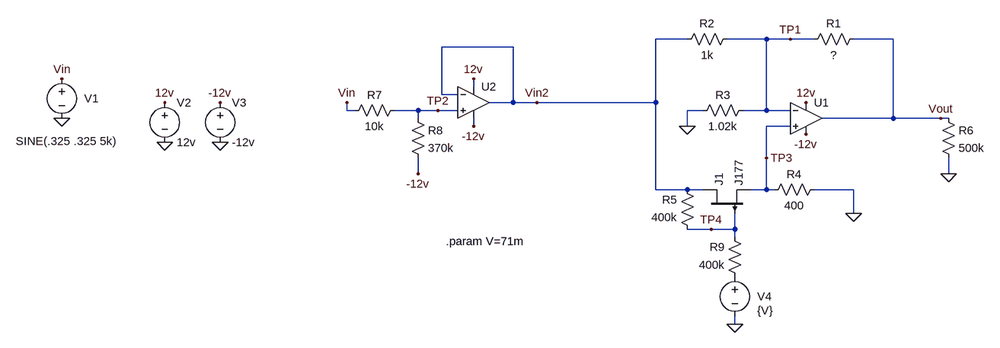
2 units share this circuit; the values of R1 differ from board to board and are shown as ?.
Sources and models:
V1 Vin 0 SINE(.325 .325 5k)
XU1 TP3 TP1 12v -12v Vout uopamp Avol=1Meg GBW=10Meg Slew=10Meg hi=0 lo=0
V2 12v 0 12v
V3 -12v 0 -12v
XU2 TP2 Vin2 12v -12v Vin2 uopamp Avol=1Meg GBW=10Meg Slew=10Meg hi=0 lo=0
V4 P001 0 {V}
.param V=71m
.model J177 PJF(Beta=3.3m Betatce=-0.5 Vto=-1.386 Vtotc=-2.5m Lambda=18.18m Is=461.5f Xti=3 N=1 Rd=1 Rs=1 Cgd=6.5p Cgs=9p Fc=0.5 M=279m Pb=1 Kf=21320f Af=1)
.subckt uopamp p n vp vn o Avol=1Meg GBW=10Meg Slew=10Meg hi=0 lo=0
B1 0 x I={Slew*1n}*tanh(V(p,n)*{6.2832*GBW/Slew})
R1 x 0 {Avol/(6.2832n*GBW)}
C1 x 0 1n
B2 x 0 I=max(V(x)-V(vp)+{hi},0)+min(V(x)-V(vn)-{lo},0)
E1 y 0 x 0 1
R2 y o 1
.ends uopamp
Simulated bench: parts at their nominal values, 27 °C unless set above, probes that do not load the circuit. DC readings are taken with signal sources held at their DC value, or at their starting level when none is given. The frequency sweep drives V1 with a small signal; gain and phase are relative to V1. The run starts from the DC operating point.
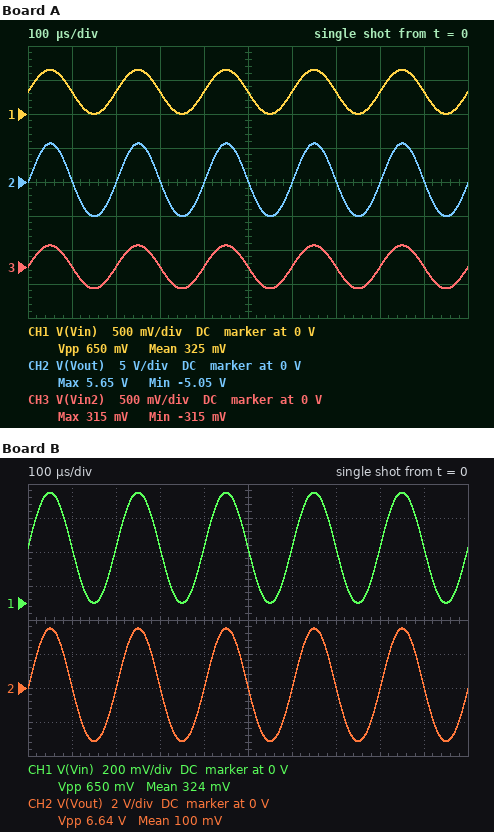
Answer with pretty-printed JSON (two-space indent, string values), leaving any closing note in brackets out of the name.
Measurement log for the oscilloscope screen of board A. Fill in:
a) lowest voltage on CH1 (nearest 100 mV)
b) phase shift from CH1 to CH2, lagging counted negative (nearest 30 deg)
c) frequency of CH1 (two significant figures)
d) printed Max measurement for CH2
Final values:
{
  "lowest voltage on CH1": "0 V",
  "phase shift from CH1 to CH2, lagging counted negative": "0 deg",
  "frequency of CH1": "5.0 kHz",
  "printed Max measurement for CH2": "5.65 V"
}
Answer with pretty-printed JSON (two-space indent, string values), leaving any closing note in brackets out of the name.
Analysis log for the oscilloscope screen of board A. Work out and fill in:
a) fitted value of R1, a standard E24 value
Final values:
{
  "fitted value of R1, a standard E24 value": "30 kΩ"
}
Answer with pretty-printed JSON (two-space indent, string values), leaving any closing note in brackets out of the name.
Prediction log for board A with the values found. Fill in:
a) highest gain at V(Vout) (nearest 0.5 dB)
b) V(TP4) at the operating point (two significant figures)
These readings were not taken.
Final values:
{
  "highest gain at V(Vout)": "24.5 dB",
  "V(TP4) at the operating point": "36 mV"
}
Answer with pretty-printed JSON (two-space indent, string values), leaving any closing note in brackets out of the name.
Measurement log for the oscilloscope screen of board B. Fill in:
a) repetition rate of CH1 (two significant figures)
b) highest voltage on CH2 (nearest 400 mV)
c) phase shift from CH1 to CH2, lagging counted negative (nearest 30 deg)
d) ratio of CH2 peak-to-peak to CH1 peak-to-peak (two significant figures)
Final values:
{
  "repetition rate of CH1": "5.0 kHz",
  "highest voltage on CH2": "3.6 V",
  "phase shift from CH1 to CH2, lagging counted negative": "0 deg",
  "ratio of CH2 peak-to-peak to CH1 peak-to-peak": "10"
}
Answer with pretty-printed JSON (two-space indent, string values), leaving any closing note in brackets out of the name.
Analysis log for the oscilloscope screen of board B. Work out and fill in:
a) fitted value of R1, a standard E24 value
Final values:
{
  "fitted value of R1, a standard E24 value": "18 kΩ"
}
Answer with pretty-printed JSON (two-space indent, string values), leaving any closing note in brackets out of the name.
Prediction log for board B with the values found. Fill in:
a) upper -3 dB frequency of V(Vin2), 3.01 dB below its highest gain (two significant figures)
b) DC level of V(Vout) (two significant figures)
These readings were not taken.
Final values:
{
  "upper -3 dB frequency of V(Vin2), 3.01 dB below its highest gain": "10 MHz",
  "DC level of V(Vout)": "6.9 mV"
}
